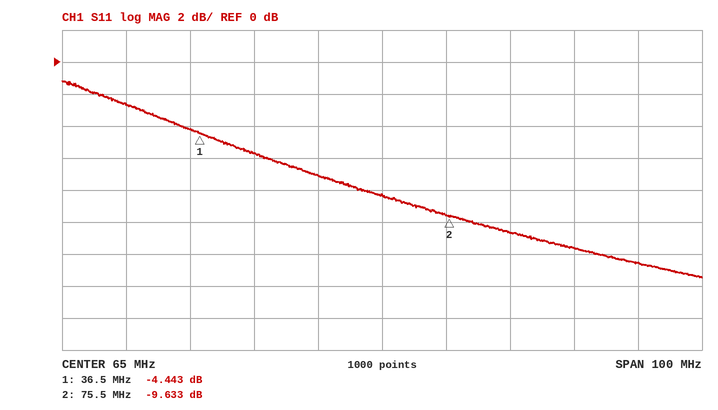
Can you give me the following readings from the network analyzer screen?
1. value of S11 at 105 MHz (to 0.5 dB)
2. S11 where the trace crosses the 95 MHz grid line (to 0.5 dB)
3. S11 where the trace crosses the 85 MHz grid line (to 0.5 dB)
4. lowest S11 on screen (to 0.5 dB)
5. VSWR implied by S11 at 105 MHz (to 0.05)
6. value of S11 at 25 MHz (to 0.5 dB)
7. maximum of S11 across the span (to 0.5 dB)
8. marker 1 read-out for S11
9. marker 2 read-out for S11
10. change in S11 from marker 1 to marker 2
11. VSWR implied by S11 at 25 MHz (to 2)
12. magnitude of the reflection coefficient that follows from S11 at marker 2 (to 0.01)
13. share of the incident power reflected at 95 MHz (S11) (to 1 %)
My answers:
-12.5 dB
-11.5 dB
-10.5 dB
-13.5 dB
1.60
-2.5 dB
-1.0 dB
-4.443 dB
-9.633 dB
-5.190 dB
6
0.33
7 %
